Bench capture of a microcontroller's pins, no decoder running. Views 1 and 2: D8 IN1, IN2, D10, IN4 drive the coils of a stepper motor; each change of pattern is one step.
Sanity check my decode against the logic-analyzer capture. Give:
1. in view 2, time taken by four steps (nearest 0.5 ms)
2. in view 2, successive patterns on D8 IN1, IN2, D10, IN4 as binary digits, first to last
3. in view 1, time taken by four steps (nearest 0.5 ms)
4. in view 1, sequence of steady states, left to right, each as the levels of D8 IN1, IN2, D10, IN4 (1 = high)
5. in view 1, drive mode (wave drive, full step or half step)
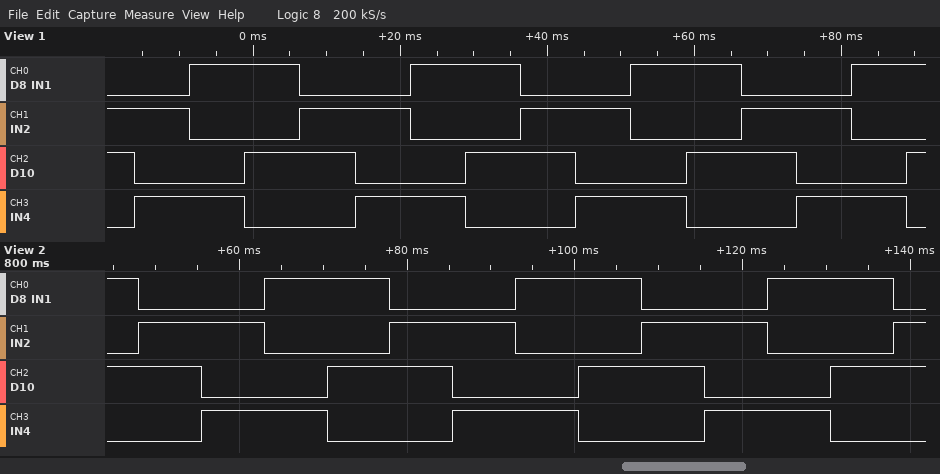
30.0 ms
1010 0110 0101 1001 1010 0110 0101 1001 1010 0110 0101 1001 1010 0110
30.0 ms
0110 0101 1001 1010 0110 0101 1001 1010 0110 0101 1001 1010 0110 0101 1001 1010
full step
